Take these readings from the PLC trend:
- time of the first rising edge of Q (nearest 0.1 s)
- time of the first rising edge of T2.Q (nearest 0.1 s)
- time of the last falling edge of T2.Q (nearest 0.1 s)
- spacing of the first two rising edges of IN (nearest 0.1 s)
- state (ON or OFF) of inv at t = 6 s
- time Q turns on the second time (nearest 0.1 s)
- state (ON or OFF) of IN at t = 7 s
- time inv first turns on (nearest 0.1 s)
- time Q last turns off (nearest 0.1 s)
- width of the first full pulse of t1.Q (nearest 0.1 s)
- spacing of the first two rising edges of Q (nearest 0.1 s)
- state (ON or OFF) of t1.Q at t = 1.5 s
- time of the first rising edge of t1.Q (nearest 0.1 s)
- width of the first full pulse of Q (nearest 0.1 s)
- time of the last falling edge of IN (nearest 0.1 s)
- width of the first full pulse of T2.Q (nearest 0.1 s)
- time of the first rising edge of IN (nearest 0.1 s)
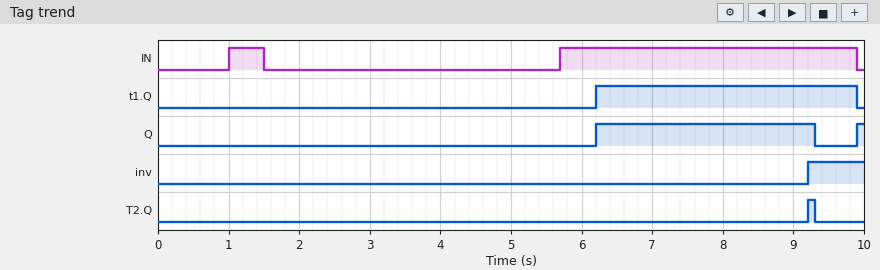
6.2 s
9.2 s
9.3 s
4.7 s
OFF
9.9 s
ON
9.2 s
9.3 s
3.7 s
3.7 s
OFF
6.2 s
3.1 s
9.9 s
0.1 s
1.0 s
